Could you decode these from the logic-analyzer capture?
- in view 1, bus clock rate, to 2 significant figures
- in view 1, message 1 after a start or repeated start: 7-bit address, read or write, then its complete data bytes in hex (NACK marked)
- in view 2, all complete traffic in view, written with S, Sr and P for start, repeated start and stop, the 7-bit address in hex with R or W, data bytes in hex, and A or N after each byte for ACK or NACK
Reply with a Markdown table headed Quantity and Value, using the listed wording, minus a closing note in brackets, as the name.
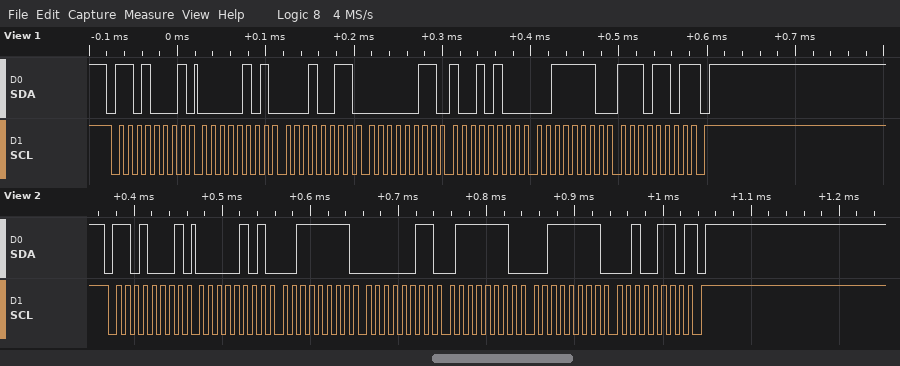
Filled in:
| Quantity | Value |
|---|---|
| in view 1, bus clock rate, to 2 significant figures | 100 kHz |
| in view 1, message 1 after a start or repeated start: 7-bit address, read or write, then its complete data bytes in hex | 0x68 read: 05 13 03 94 3E ED NACK |
| in view 2, all complete traffic in view, written with S, Sr and P for start, repeated start and stop, the 7-bit address in hex with R or W, data bytes in hex, and A or N after each byte for ACK or NACK | S 68R A 05 A 3F A 03 A 7E A 3F A 26 N P |
